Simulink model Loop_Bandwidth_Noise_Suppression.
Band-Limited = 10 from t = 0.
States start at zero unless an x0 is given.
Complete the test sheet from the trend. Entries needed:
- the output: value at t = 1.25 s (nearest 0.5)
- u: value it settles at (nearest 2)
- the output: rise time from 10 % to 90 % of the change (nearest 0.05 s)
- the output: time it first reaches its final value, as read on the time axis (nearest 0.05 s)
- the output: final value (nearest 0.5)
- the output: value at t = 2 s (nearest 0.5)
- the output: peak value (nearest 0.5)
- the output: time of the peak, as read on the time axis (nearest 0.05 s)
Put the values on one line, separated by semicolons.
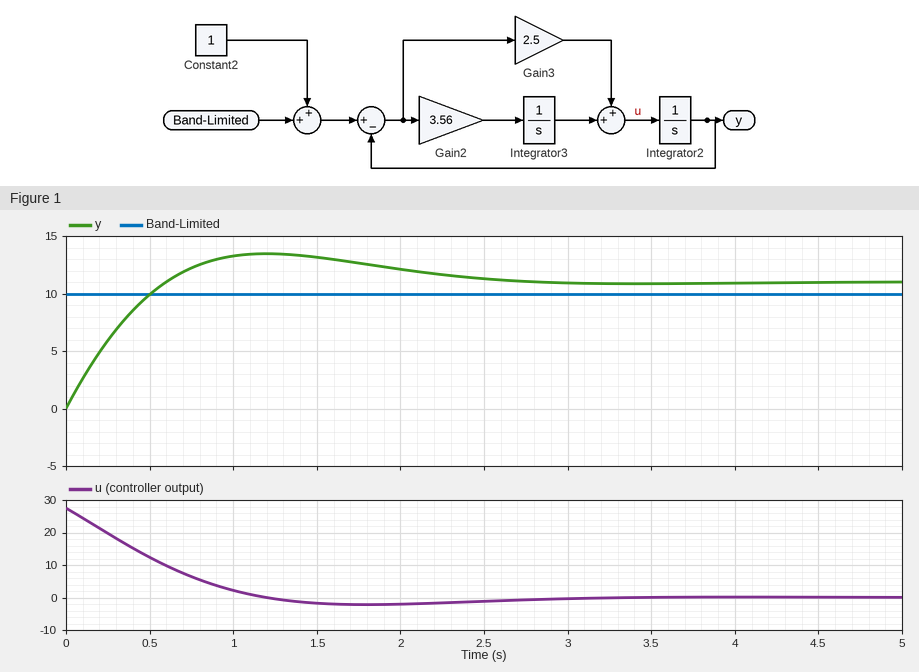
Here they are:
13.5; 0; 0.45 s; 0.60 s; 11.0; 12.0; 13.5; 1.20 s
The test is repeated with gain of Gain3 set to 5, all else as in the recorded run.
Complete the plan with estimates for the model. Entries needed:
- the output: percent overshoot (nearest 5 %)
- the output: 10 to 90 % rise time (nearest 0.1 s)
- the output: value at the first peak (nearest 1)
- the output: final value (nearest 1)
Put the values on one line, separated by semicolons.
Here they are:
10 %; 0.3 s; 12; 11
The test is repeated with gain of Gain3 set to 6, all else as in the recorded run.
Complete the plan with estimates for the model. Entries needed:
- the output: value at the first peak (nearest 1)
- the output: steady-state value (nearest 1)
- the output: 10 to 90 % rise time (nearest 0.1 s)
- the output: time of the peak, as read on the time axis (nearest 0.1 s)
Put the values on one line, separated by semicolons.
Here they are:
12; 11; 0.3 s; 0.9 s
